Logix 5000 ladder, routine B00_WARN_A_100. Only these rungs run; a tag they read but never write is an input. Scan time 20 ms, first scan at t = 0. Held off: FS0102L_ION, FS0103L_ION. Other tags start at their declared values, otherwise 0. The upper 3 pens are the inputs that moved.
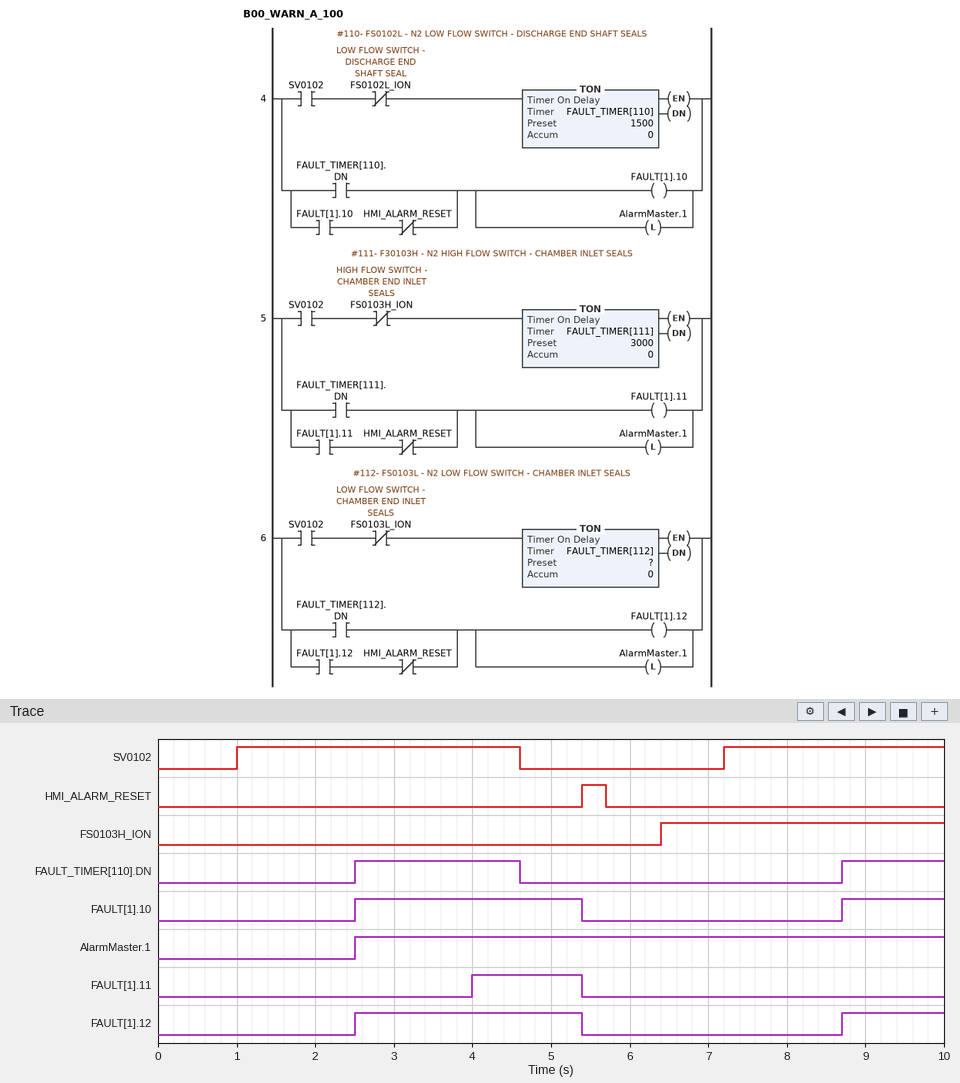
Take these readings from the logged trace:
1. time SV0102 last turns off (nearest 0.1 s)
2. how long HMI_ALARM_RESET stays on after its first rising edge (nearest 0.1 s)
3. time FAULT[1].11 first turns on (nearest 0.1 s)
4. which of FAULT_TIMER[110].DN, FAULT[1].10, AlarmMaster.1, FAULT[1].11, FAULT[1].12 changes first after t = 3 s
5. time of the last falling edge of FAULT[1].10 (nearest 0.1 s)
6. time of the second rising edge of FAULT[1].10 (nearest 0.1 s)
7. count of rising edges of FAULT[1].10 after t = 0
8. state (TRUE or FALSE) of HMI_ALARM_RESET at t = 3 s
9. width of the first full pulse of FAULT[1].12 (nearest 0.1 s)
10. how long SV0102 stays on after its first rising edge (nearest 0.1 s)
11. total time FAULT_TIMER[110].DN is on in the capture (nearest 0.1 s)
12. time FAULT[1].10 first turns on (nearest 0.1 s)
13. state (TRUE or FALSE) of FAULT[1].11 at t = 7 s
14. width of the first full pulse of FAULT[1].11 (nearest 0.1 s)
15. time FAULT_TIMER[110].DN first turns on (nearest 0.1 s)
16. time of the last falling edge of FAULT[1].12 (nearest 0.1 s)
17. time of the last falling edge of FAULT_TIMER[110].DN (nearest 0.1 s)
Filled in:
4.6 s
0.3 s
4.0 s
FAULT[1].11
5.4 s
8.7 s
2
FALSE
2.9 s
3.6 s
3.4 s
2.5 s
FALSE
1.4 s
2.5 s
5.4 s
4.6 s
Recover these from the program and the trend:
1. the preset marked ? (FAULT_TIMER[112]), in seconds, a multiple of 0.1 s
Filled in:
1.5 s
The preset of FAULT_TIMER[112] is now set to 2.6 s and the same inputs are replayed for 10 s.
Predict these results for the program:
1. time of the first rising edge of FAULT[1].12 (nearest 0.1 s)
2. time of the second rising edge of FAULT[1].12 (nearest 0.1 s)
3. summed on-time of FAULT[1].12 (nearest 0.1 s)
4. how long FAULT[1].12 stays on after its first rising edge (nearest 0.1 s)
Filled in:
3.6 s
9.8 s
2.0 s
1.8 s
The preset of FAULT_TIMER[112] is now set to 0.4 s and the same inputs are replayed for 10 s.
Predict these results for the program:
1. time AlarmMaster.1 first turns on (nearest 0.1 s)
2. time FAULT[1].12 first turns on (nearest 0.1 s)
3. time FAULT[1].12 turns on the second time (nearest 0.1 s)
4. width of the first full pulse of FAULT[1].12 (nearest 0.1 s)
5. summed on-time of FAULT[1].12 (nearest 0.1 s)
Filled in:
1.4 s
1.4 s
7.6 s
4.0 s
6.4 s
